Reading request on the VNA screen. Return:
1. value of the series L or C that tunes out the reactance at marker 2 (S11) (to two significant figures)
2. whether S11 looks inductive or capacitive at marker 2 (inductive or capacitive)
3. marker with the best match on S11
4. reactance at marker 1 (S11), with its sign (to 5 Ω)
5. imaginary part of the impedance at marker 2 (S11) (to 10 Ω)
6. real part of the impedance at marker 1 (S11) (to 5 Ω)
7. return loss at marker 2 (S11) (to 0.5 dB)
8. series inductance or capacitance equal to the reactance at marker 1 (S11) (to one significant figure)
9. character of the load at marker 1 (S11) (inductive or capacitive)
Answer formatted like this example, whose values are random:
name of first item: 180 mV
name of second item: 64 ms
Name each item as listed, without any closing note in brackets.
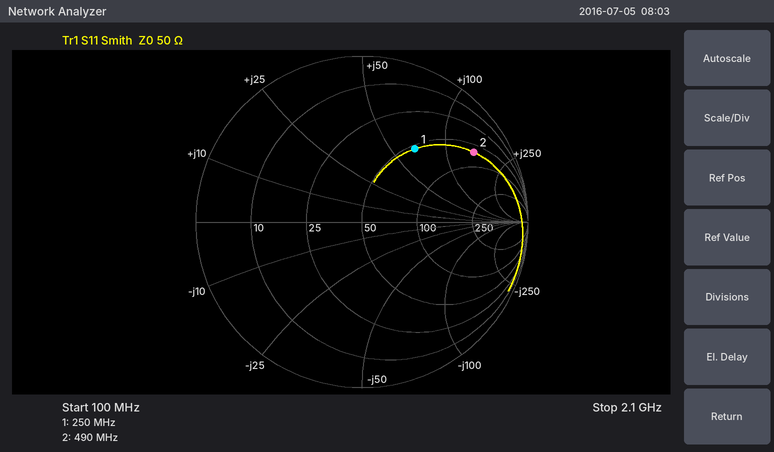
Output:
value of the series L or C that tunes out the reactance at marker 2 (S11): 2.2 pF
whether S11 looks inductive or capacitive at marker 2: inductive
marker with the best match on S11: marker 1
reactance at marker 1 (S11), with its sign: +65 Ω
imaginary part of the impedance at marker 2 (S11): +150 Ω
real part of the impedance at marker 1 (S11): 55 Ω
return loss at marker 2 (S11): 2.0 dB
series inductance or capacitance equal to the reactance at marker 1 (S11): 40 nH
character of the load at marker 1 (S11): inductive
